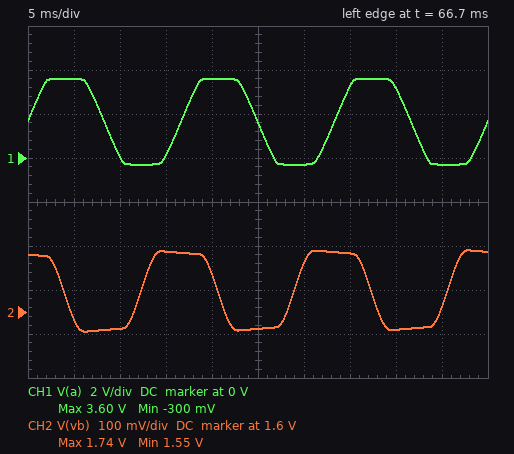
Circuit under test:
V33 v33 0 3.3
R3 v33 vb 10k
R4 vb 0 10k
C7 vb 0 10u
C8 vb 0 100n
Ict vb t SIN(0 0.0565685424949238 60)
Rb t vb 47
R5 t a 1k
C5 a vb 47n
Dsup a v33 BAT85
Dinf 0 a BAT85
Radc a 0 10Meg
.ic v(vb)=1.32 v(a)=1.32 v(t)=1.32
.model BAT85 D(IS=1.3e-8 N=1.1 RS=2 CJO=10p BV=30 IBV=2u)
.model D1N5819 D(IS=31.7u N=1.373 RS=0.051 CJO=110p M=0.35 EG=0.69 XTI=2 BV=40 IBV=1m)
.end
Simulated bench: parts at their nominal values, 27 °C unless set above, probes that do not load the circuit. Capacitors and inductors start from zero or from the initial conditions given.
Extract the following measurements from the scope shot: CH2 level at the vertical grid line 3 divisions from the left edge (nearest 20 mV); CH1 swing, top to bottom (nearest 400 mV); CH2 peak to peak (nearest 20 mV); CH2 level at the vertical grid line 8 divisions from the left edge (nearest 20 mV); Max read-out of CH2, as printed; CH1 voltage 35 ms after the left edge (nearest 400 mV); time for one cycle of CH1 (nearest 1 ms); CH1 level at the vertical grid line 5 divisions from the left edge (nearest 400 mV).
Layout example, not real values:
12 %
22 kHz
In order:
1.74 V
4.0 V
180 mV
1.56 V
1.74 V
3.2 V
17 ms
1.6 V
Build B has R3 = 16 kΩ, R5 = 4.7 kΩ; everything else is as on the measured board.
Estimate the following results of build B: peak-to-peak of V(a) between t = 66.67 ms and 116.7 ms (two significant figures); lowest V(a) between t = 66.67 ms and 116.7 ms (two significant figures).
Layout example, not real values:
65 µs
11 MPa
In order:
3.8 V
-280 mV
